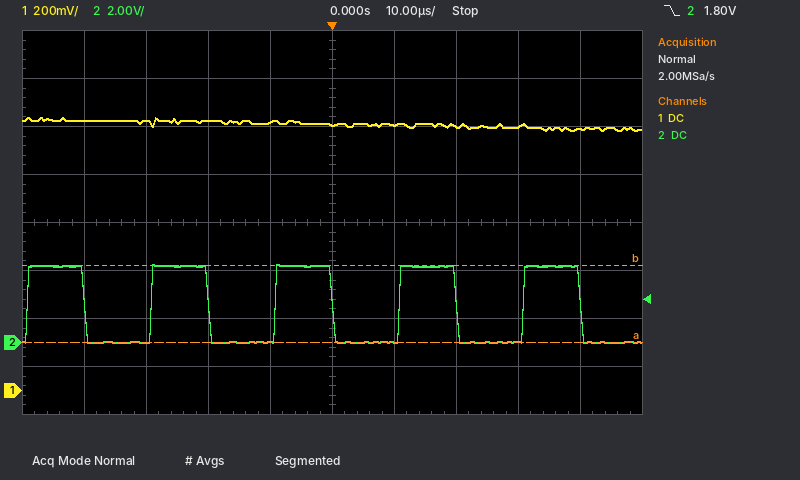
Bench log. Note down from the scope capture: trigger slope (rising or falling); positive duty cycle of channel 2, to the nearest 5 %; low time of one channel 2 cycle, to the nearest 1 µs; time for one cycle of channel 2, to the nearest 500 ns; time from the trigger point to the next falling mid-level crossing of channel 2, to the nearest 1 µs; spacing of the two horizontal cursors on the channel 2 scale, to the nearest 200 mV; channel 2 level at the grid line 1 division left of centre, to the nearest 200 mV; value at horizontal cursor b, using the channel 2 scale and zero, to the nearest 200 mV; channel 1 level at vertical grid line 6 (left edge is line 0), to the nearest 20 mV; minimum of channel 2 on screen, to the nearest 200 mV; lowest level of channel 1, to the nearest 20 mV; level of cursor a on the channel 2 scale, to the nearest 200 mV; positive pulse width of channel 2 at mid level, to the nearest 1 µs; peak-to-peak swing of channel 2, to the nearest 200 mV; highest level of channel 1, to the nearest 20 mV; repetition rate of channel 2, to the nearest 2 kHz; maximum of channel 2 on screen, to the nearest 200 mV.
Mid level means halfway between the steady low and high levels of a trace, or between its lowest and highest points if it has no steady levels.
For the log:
falling
45 %
11 µs
20.0 µs
20 µs
3.2 V
0.0 V
3.2 V
1.10 V
0.0 V
1.08 V
0.0 V
9 µs
3.2 V
1.14 V
50 kHz
3.2 V
